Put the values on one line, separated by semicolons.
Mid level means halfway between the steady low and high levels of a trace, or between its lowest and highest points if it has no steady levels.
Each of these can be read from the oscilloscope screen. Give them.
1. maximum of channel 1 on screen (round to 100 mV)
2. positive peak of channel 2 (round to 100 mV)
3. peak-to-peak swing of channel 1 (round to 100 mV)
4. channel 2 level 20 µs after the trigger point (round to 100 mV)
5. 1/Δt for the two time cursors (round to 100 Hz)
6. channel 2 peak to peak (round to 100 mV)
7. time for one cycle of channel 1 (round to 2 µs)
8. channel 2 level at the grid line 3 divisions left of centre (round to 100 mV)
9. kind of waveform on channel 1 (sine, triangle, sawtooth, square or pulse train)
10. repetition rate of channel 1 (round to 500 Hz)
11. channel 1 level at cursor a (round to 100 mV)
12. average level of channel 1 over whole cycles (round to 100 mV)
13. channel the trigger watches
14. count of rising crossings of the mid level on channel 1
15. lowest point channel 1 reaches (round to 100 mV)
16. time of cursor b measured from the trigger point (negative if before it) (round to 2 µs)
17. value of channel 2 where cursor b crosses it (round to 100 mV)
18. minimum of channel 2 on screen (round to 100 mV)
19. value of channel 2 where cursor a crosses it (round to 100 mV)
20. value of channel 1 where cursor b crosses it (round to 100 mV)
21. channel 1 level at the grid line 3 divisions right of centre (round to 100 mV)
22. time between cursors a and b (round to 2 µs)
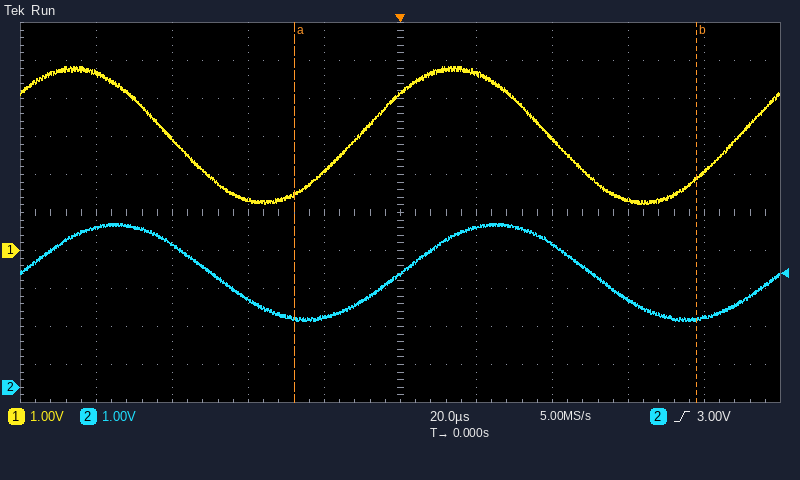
4.8 V; 4.3 V; 3.6 V; 4.2 V; 9.4 kHz; 2.6 V; 100 µs; 3.7 V; sine; 10.0 kHz; 1.5 V; 3.0 V; channel 2; 2; 1.2 V; +78 µs; 1.8 V; 1.7 V; 1.8 V; 1.9 V; 1.3 V; 106 µs
